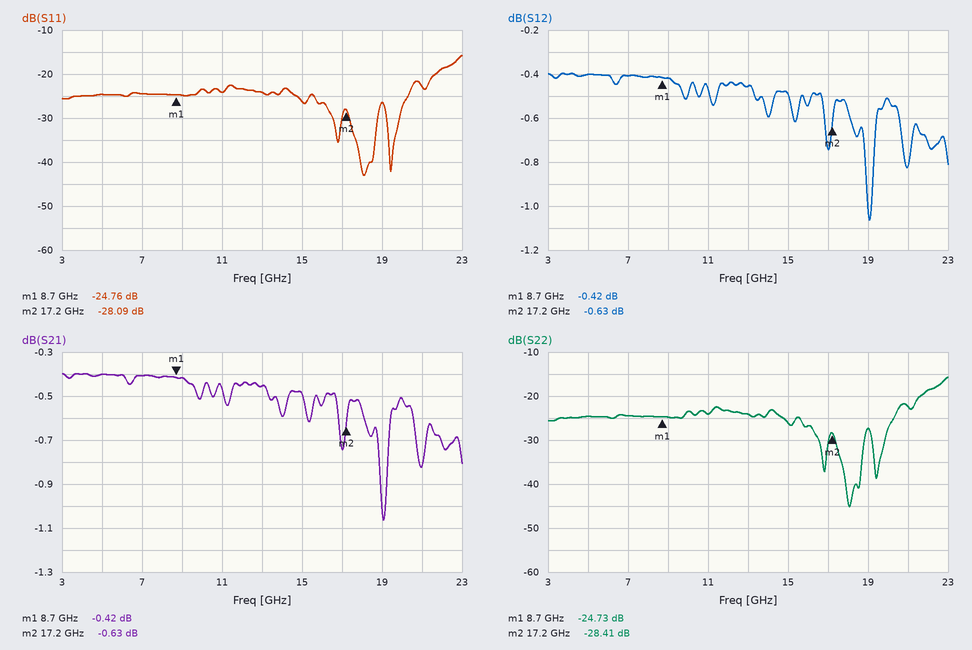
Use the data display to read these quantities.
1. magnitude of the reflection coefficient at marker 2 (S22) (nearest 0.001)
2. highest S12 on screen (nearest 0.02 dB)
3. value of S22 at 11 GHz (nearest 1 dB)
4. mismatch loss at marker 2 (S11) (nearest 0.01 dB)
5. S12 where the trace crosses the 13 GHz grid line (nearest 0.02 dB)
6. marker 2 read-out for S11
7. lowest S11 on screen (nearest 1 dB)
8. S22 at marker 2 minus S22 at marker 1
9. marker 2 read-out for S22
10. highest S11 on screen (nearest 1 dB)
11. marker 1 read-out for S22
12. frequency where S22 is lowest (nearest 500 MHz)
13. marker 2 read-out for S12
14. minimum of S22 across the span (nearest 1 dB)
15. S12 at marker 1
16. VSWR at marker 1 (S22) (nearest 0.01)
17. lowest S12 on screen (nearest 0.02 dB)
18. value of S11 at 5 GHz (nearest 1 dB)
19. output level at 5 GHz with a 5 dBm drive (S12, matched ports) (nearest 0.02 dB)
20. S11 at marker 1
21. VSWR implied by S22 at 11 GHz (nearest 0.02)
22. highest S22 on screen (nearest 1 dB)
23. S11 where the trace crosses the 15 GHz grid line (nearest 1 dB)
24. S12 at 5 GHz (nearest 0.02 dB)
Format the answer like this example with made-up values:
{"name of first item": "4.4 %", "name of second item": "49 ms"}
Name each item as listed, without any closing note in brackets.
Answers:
{"magnitude of the reflection coefficient at marker 2 (S22)": "0.038", "highest S12 on screen": "-0.40 dB", "value of S22 at 11 GHz": "-24 dB", "mismatch loss at marker 2 (S11)": "0.01 dB", "S12 where the trace crosses the 13 GHz grid line": "-0.46 dB", "marker 2 read-out for S11": "-28.09 dB", "lowest S11 on screen": "-43 dB", "S22 at marker 2 minus S22 at marker 1": "-3.68 dB", "marker 2 read-out for S22": "-28.41 dB", "highest S11 on screen": "-16 dB", "marker 1 read-out for S22": "-24.73 dB", "frequency where S22 is lowest": "18.0 GHz", "marker 2 read-out for S12": "-0.63 dB", "minimum of S22 across the span": "-45 dB", "S12 at marker 1": "-0.42 dB", "VSWR at marker 1 (S22)": "1.12", "lowest S12 on screen": "-1.06 dB", "value of S11 at 5 GHz": "-25 dB", "output level at 5 GHz with a 5 dBm drive (S12, matched ports)": "4.60 dBm", "S11 at marker 1": "-24.76 dB", "VSWR implied by S22 at 11 GHz": "1.14", "highest S22 on screen": "-16 dB", "S11 where the trace crosses the 15 GHz grid line": "-26 dB", "S12 at 5 GHz": "-0.40 dB"}
